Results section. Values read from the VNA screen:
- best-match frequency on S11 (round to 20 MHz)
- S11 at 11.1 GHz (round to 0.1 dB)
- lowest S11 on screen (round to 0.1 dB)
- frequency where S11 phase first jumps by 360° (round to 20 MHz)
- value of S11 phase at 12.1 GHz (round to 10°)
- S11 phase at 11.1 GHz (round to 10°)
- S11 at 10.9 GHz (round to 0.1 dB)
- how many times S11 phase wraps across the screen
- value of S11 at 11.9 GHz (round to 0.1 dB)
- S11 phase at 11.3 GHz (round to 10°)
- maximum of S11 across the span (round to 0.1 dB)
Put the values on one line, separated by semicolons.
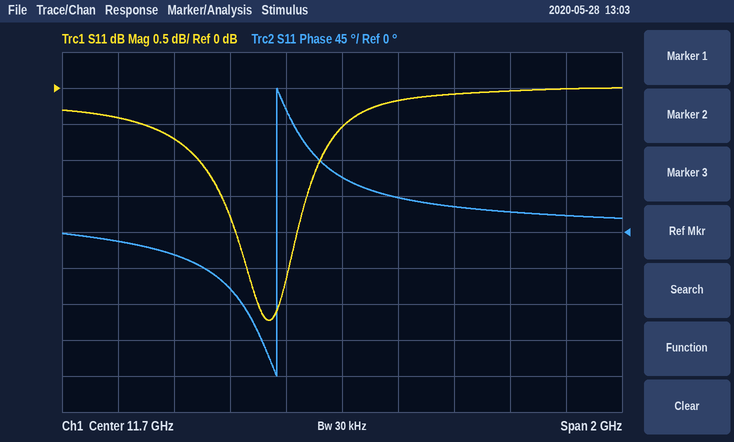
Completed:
11.44 GHz; -0.7 dB; -3.2 dB; 11.46 GHz; 30°; -30°; -0.4 dB; 1; -0.2 dB; -70°; 0.0 dB
